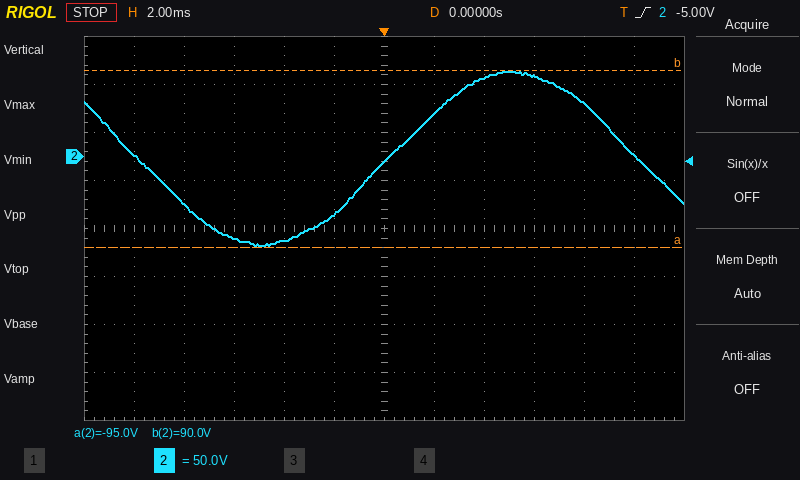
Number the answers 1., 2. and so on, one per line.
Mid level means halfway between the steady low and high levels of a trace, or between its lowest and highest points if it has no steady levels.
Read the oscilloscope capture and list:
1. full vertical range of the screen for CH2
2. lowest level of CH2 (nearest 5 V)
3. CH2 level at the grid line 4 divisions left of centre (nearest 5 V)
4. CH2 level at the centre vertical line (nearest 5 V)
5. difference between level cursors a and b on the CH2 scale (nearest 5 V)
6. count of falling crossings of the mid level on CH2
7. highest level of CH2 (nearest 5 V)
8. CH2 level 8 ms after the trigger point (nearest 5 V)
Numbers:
1. 400 V
2. -95 V
3. -50 V
4. -5 V
5. 185 V
6. 2
7. 90 V
8. 55 V
